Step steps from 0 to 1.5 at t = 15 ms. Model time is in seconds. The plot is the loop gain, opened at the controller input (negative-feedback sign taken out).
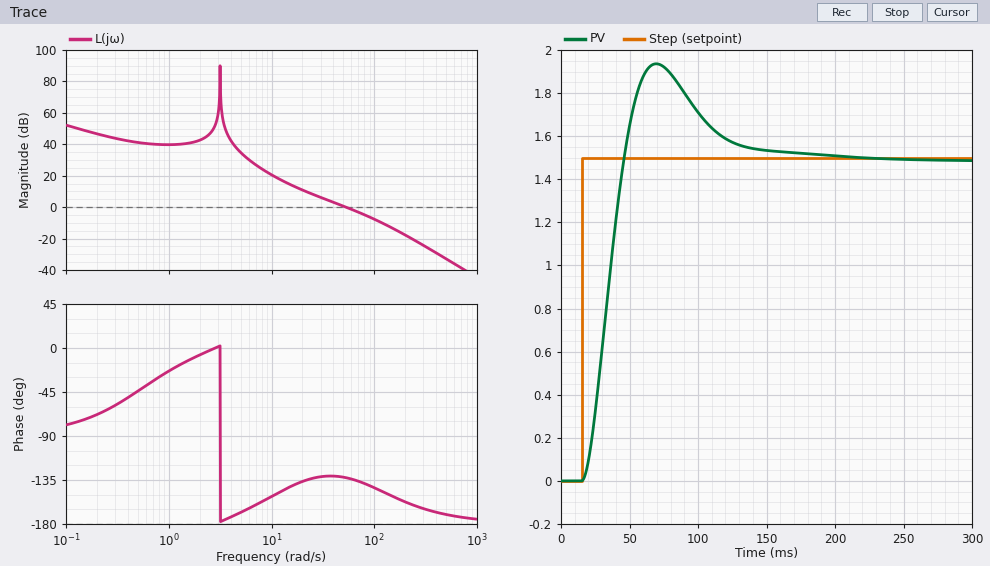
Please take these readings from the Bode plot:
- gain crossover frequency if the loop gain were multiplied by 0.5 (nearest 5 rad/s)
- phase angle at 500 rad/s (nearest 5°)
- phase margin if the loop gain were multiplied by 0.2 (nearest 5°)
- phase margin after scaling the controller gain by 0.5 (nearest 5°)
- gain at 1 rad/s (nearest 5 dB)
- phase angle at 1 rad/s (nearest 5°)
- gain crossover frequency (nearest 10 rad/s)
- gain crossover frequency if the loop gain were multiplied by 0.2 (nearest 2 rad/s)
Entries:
30 rad/s
-170°
40°
50°
40 dB
-25°
50 rad/s
16 rad/s
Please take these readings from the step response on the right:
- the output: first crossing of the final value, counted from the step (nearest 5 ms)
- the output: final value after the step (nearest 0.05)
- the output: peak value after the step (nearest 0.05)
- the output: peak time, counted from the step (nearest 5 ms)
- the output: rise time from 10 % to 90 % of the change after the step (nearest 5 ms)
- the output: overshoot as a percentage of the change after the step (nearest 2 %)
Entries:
30 ms
1.50
1.95
55 ms
20 ms
30 %
